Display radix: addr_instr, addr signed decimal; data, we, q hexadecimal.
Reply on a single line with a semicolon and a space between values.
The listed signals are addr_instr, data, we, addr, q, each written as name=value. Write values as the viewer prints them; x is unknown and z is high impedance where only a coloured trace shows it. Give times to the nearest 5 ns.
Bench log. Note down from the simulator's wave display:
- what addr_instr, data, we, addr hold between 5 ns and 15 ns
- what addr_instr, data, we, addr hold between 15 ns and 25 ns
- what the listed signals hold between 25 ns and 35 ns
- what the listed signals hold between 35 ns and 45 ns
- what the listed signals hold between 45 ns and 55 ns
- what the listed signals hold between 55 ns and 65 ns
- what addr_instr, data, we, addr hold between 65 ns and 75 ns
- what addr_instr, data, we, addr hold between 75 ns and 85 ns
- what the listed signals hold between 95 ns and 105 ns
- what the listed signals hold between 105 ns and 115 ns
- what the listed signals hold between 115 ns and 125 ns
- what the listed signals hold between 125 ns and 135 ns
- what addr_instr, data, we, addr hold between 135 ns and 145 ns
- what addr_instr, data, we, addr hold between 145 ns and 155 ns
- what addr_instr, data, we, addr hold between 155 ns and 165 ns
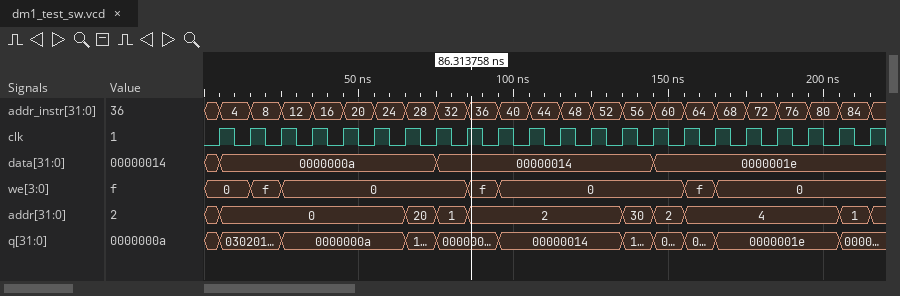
addr_instr=4, data=0000000a, we=0, addr=0; addr_instr=8, data=0000000a, we=f, addr=0; addr_instr=12, data=0000000a, we=0, addr=0, q=0000000a; addr_instr=16, data=0000000a, we=0, addr=0, q=0000000a; addr_instr=20, data=0000000a, we=0, addr=0, q=0000000a; addr_instr=24, data=0000000a, we=0, addr=0, q=0000000a; addr_instr=28, data=0000000a, we=0, addr=20; addr_instr=32, data=00000014, we=0, addr=1; addr_instr=40, data=00000014, we=0, addr=2, q=00000014; addr_instr=44, data=00000014, we=0, addr=2, q=00000014; addr_instr=48, data=00000014, we=0, addr=2, q=00000014; addr_instr=52, data=00000014, we=0, addr=2, q=00000014; addr_instr=56, data=00000014, we=0, addr=30; addr_instr=60, data=0000001e, we=0, addr=2; addr_instr=64, data=0000001e, we=f, addr=4
